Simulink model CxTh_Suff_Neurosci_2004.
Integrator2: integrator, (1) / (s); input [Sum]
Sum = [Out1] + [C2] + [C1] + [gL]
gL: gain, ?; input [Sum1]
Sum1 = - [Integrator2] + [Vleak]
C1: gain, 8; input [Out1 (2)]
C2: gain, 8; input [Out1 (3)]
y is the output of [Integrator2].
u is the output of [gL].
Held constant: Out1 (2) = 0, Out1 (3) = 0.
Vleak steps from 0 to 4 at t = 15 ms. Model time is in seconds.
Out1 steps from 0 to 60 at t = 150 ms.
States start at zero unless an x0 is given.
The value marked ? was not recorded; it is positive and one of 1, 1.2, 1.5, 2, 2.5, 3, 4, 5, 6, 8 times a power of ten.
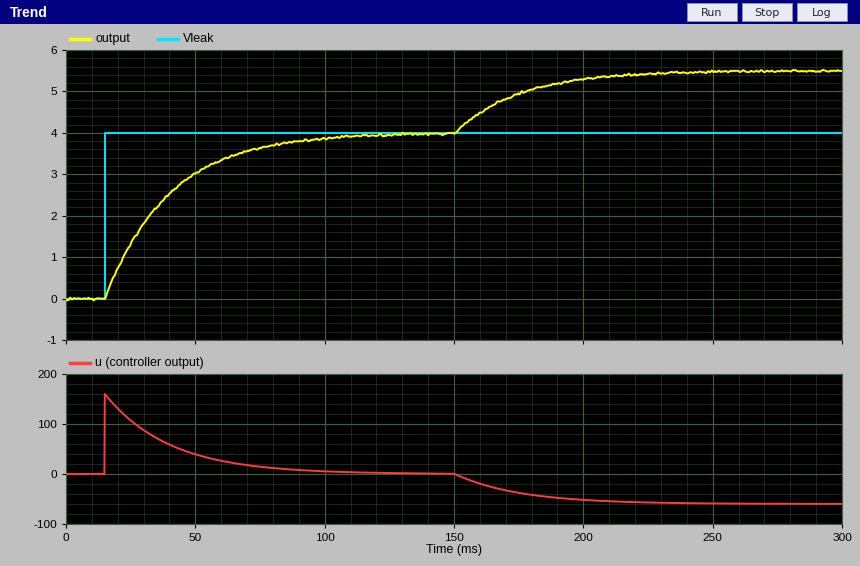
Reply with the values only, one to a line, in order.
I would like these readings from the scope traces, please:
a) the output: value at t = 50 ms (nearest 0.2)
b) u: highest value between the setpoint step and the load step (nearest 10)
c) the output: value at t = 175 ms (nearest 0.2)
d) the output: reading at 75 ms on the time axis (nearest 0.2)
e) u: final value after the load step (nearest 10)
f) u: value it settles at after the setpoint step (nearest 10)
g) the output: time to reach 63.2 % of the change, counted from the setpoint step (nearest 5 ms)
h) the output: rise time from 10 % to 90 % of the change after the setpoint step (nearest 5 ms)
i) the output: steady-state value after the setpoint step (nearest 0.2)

3.0
160
5.0
3.6
-60
0
25 ms
55 ms
4.0
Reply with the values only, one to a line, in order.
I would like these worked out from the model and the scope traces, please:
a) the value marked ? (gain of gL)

40
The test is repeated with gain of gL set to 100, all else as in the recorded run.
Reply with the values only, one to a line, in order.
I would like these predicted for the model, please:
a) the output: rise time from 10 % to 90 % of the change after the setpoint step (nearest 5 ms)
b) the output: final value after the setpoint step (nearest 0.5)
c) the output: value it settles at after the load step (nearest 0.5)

20 ms
4.0
4.5
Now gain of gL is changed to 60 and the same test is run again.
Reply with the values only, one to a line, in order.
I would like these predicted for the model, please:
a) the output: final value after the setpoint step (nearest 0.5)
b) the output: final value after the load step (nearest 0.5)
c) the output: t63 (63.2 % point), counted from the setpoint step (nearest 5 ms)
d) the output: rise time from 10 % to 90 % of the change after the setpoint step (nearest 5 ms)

4.0
5.0
15 ms
35 ms
